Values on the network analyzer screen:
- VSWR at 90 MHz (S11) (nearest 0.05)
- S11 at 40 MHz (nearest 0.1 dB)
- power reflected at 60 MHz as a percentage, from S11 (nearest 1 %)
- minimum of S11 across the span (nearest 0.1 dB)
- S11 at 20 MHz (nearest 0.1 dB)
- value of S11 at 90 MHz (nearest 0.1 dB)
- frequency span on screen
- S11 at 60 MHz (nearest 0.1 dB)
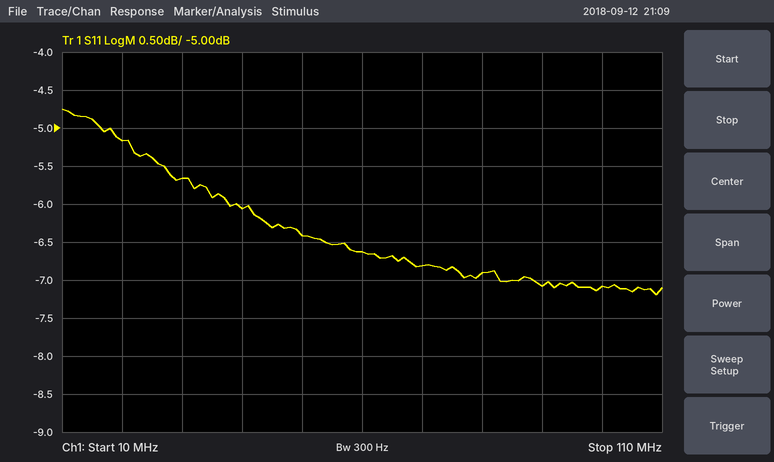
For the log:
2.60
-6.1 dB
22 %
-7.2 dB
-5.2 dB
-7.1 dB
100 MHz
-6.6 dB
